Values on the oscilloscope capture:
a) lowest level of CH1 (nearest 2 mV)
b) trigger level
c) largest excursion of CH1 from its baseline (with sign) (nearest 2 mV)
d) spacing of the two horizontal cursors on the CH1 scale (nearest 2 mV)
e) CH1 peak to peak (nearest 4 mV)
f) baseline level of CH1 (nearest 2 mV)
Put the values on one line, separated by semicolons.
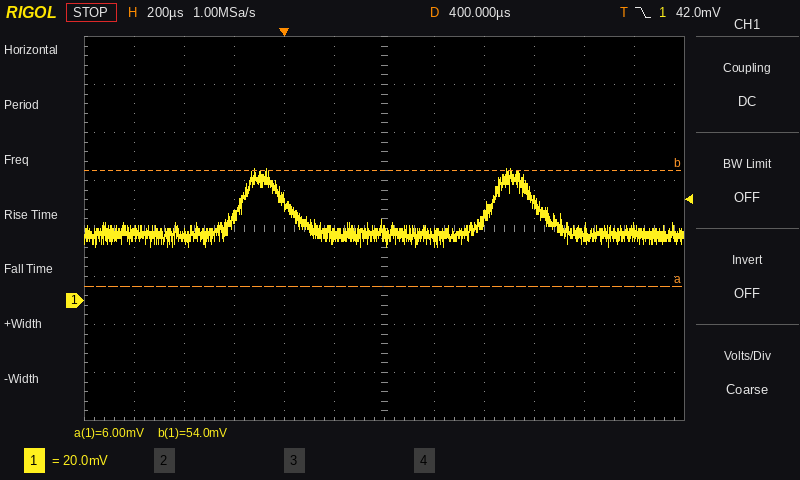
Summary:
22 mV; 42.0 mV; +28 mV; 48 mV; 32 mV; 28 mV
